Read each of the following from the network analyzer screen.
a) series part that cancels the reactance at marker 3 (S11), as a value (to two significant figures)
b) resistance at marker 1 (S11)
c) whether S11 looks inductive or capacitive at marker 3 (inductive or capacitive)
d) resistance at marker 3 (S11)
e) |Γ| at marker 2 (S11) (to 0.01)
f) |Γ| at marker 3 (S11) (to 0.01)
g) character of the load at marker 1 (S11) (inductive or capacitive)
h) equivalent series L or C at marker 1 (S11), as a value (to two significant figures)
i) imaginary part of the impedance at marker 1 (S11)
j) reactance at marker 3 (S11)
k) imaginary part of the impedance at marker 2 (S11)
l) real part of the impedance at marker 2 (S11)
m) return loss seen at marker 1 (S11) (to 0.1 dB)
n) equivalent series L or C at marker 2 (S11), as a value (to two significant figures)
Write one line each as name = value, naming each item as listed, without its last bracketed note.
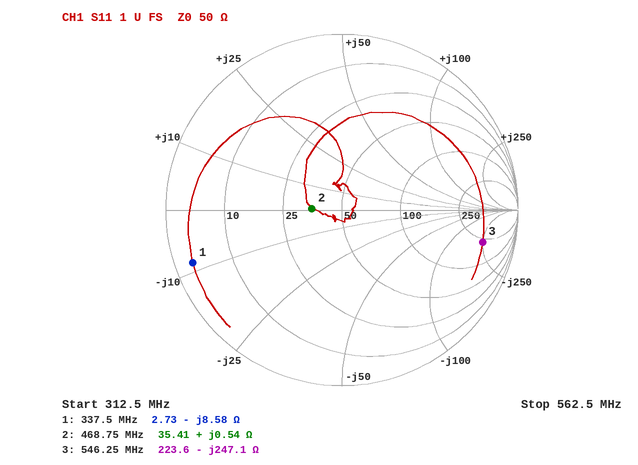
series part that cancels the reactance at marker 3 (S11), as a value = 72 nH
resistance at marker 1 = 2.73 Ω
whether S11 looks inductive or capacitive at marker 3 = capacitive
resistance at marker 3 = 223.6 Ω
|Γ| at marker 2 (S11) = 0.17
|Γ| at marker 3 (S11) = 0.82
character of the load at marker 1 (S11) = capacitive
equivalent series L or C at marker 1 (S11), as a value = 55 pF
imaginary part of the impedance at marker 1 = -8.58 Ω
reactance at marker 3 = -247.1 Ω
imaginary part of the impedance at marker 2 = +0.54 Ω
real part of the impedance at marker 2 = 35.41 Ω
return loss seen at marker 1 (S11) = 0.9 dB
equivalent series L or C at marker 2 (S11), as a value = 180 pH
